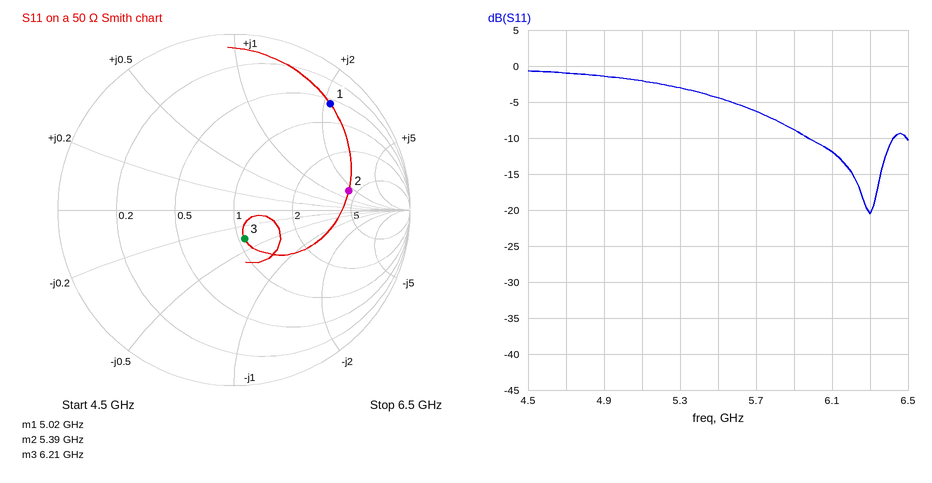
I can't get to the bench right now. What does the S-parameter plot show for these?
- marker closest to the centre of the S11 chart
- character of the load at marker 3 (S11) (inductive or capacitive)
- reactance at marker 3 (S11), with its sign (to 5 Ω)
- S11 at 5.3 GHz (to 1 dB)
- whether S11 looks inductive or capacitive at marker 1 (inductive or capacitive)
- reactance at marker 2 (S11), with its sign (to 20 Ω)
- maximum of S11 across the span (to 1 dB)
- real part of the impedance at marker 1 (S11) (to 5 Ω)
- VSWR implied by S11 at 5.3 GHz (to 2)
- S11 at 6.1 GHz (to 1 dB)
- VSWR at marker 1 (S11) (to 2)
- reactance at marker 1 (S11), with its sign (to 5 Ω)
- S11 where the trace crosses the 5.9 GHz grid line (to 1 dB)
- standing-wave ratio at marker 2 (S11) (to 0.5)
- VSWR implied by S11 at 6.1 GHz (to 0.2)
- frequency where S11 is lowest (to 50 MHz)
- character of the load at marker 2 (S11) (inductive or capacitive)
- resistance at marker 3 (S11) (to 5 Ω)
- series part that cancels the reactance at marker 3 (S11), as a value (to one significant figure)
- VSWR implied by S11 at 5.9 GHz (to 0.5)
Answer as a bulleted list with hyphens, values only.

- marker 3
- capacitive
- -20 Ω
- -3 dB
- inductive
- +80 Ω
- -1 dB
- 30 Ω
- 6
- -12 dB
- 10
- +105 Ω
- -9 dB
- 5.0
- 1.6
- 6.30 GHz
- inductive
- 55 Ω
- 500 pH
- 2.0
